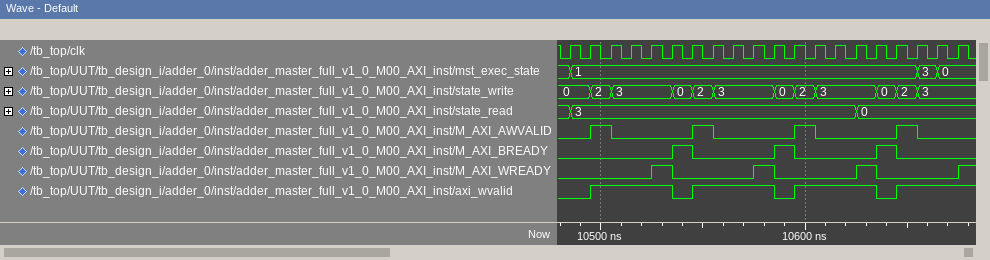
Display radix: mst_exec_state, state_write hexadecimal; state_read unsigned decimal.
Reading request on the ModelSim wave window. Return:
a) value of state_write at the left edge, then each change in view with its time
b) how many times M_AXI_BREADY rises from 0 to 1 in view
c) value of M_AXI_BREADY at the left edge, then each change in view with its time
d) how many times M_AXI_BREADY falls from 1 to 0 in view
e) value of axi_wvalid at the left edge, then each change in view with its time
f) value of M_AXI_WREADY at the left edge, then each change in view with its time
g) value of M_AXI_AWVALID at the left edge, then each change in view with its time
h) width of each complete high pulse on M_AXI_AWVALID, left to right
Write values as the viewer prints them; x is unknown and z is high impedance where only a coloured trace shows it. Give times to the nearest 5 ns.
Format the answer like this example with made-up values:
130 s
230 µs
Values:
0, 2 at 10495 ns, 3 at 10505 ns, 0 at 10535 ns, 2 at 10545 ns, 3 at 10555 ns, 0 at 10585 ns, 2 at 10595 ns, 3 at 10605 ns, 0 at 10635 ns, 2 at 10645 ns, 3 at 10655 ns
3
0, 1 at 10535 ns, 0 at 10545 ns, 1 at 10585 ns, 0 at 10595 ns, 1 at 10635 ns, 0 at 10645 ns
3
0, 1 at 10495 ns, 0 at 10535 ns, 1 at 10545 ns, 0 at 10585 ns, 1 at 10595 ns, 0 at 10635 ns, 1 at 10645 ns
0, 1 at 10525 ns, 0 at 10535 ns, 1 at 10575 ns, 0 at 10585 ns, 1 at 10625 ns, 0 at 10635 ns, 1 at 10675 ns
0, 1 at 10495 ns, 0 at 10505 ns, 1 at 10545 ns, 0 at 10555 ns, 1 at 10595 ns, 0 at 10605 ns, 1 at 10645 ns, 0 at 10655 ns
10 ns, 10 ns, 10 ns, 10 ns
